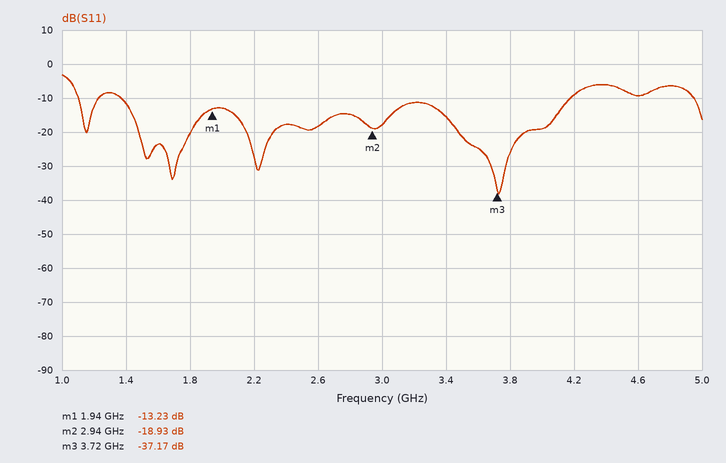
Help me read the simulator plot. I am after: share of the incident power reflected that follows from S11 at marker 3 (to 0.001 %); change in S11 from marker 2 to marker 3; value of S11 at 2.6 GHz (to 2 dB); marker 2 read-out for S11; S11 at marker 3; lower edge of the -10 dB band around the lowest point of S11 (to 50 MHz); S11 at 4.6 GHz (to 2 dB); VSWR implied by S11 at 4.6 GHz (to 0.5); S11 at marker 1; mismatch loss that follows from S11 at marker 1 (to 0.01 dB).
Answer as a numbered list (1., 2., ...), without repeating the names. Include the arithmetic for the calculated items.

1. 10^(-37.17/10) ≈ 0.019 %
2. -37.17 − (-18.93) = -18.24 dB
3. -18 dB
4. -18.93 dB
5. -37.17 dB
6. 1.35 GHz
7. -10 dB
8. |Γ| = 10^(-10/20) = 0.3162; VSWR = (1 + 0.3162)/(1 − 0.3162) ≈ 1.92, so 2.0 to the nearest 0.5
9. -13.23 dB
10. −10 log10(1 − 10^(-13.23/10)) ≈ 0.21 dB
